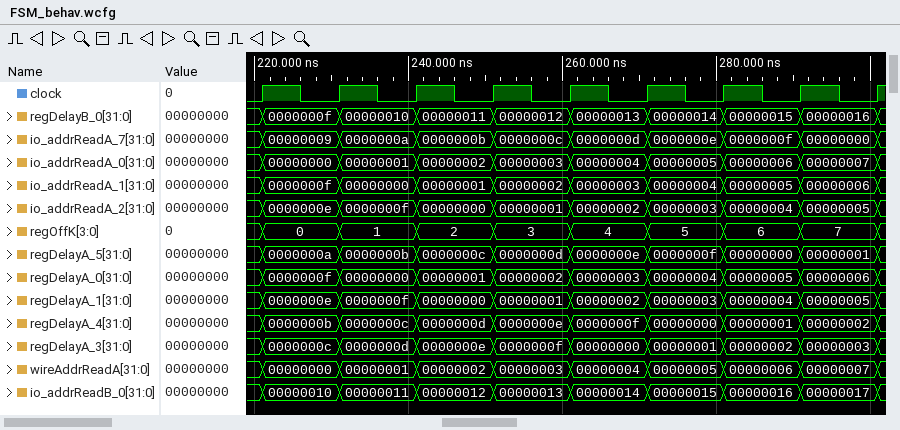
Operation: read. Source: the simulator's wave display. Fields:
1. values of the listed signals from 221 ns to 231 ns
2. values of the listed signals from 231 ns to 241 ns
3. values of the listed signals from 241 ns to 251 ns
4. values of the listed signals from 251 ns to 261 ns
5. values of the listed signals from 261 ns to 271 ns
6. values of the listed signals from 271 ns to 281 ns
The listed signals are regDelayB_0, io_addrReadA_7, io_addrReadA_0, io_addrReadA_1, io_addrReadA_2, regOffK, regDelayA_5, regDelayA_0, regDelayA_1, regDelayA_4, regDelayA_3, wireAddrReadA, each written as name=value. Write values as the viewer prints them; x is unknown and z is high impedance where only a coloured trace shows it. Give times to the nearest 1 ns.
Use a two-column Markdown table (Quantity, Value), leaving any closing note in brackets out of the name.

| Quantity | Value |
|---|---|
| values of the listed signals from 221 ns to 231 ns | regDelayB_0=0000000f, io_addrReadA_7=00000009, io_addrReadA_0=00000000, io_addrReadA_1=0000000f, io_addrReadA_2=0000000e, regOffK=0, regDelayA_5=0000000a, regDelayA_0=0000000f, regDelayA_1=0000000e, regDelayA_4=0000000b, regDelayA_3=0000000c, wireAddrReadA=00000000 |
| values of the listed signals from 231 ns to 241 ns | regDelayB_0=00000010, io_addrReadA_7=0000000a, io_addrReadA_0=00000001, io_addrReadA_1=00000000, io_addrReadA_2=0000000f, regOffK=1, regDelayA_5=0000000b, regDelayA_0=00000000, regDelayA_1=0000000f, regDelayA_4=0000000c, regDelayA_3=0000000d, wireAddrReadA=00000001 |
| values of the listed signals from 241 ns to 251 ns | regDelayB_0=00000011, io_addrReadA_7=0000000b, io_addrReadA_0=00000002, io_addrReadA_1=00000001, io_addrReadA_2=00000000, regOffK=2, regDelayA_5=0000000c, regDelayA_0=00000001, regDelayA_1=00000000, regDelayA_4=0000000d, regDelayA_3=0000000e, wireAddrReadA=00000002 |
| values of the listed signals from 251 ns to 261 ns | regDelayB_0=00000012, io_addrReadA_7=0000000c, io_addrReadA_0=00000003, io_addrReadA_1=00000002, io_addrReadA_2=00000001, regOffK=3, regDelayA_5=0000000d, regDelayA_0=00000002, regDelayA_1=00000001, regDelayA_4=0000000e, regDelayA_3=0000000f, wireAddrReadA=00000003 |
| values of the listed signals from 261 ns to 271 ns | regDelayB_0=00000013, io_addrReadA_7=0000000d, io_addrReadA_0=00000004, io_addrReadA_1=00000003, io_addrReadA_2=00000002, regOffK=4, regDelayA_5=0000000e, regDelayA_0=00000003, regDelayA_1=00000002, regDelayA_4=0000000f, regDelayA_3=00000000, wireAddrReadA=00000004 |
| values of the listed signals from 271 ns to 281 ns | regDelayB_0=00000014, io_addrReadA_7=0000000e, io_addrReadA_0=00000005, io_addrReadA_1=00000004, io_addrReadA_2=00000003, regOffK=5, regDelayA_5=0000000f, regDelayA_0=00000004, regDelayA_1=00000003, regDelayA_4=00000000, regDelayA_3=00000001, wireAddrReadA=00000005 |
